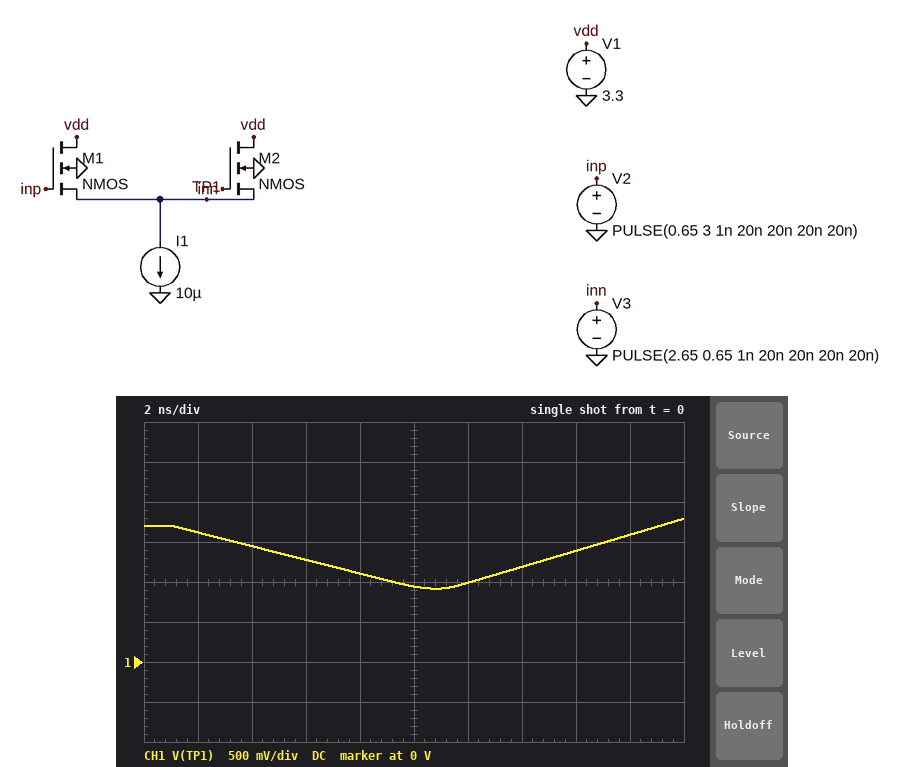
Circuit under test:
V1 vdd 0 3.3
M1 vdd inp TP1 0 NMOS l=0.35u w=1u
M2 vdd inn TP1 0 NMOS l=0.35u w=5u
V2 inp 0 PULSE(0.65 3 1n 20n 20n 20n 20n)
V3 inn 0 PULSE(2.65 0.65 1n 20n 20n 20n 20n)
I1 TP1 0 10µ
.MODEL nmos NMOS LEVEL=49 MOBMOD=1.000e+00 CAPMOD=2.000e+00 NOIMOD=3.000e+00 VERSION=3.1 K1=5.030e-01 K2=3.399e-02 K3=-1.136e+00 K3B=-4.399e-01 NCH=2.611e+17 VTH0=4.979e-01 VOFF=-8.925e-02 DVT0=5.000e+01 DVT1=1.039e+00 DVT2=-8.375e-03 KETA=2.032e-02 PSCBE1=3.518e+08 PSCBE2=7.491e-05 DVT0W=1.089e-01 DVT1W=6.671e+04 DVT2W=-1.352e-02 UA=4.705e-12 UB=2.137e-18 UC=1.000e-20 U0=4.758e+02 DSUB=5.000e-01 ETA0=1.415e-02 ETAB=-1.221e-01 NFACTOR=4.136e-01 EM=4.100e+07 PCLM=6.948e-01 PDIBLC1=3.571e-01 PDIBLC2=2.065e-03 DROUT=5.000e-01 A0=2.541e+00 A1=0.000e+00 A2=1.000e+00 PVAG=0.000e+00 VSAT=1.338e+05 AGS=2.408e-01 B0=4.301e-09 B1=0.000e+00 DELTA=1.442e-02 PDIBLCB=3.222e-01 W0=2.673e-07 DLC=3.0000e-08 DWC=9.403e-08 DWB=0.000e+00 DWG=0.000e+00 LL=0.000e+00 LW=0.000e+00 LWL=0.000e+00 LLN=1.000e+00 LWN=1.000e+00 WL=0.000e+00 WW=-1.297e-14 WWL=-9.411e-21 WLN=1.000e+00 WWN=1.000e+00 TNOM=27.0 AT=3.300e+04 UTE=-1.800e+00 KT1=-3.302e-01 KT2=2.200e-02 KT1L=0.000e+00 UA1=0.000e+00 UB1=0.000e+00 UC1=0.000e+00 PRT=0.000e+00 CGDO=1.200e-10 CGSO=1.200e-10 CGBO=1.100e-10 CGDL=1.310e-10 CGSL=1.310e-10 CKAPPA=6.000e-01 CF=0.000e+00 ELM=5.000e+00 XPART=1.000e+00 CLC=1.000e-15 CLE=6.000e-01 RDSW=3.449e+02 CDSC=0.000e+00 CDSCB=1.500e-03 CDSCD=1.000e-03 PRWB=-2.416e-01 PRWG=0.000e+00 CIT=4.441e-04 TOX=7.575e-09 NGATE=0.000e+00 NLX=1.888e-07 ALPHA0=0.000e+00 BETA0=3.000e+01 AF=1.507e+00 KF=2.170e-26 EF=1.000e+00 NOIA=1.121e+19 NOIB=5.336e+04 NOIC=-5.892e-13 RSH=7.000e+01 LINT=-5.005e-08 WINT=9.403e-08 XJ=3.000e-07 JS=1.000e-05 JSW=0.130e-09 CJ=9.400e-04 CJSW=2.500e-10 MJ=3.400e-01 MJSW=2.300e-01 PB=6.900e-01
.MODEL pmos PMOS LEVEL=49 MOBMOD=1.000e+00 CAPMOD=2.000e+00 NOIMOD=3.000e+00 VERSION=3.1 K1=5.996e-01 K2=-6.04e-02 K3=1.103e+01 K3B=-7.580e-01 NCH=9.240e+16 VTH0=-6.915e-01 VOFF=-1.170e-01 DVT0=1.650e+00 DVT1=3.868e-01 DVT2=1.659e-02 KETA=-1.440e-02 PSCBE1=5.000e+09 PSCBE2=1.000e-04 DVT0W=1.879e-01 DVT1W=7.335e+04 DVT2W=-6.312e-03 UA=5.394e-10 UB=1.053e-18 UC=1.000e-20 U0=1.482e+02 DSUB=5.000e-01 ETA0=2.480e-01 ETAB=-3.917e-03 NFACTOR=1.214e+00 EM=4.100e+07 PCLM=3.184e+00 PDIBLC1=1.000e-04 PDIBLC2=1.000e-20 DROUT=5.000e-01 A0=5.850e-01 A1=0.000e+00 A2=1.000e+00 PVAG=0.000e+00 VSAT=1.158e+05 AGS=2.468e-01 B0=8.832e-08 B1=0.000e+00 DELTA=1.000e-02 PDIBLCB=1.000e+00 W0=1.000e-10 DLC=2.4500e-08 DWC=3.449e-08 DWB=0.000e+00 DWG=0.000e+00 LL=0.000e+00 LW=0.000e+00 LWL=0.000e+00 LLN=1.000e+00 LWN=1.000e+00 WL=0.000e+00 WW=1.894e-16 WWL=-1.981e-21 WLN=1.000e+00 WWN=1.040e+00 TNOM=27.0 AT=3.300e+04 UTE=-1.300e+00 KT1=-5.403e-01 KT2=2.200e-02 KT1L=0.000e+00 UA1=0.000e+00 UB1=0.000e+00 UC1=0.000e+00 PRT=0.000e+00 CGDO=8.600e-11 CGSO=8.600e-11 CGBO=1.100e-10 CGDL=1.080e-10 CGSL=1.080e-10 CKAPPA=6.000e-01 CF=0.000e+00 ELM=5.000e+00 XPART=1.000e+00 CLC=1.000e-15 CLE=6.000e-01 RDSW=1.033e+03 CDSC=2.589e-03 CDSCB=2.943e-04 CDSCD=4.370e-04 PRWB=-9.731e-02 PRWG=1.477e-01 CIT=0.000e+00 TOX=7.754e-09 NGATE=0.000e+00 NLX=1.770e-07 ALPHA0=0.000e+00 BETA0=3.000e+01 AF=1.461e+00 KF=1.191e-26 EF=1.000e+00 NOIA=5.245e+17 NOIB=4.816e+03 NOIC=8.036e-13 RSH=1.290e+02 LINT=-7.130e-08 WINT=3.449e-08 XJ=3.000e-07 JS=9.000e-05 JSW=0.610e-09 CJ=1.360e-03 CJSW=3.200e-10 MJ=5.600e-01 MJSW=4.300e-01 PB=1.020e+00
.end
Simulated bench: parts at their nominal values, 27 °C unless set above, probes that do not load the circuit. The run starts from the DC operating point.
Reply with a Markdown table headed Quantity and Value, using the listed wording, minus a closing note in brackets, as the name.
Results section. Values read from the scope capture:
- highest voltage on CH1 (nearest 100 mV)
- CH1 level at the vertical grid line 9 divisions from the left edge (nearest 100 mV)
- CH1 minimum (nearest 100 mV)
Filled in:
| Quantity | Value |
|---|---|
| highest voltage on CH1 | 1.8 V |
| CH1 level at the vertical grid line 9 divisions from the left edge | 1.6 V |
| CH1 minimum | 900 mV |
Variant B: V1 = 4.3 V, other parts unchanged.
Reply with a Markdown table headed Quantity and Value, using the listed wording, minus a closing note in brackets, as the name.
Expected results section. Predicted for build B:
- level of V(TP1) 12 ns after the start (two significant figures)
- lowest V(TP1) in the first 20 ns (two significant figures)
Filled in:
| Quantity | Value |
|---|---|
| level of V(TP1) 12 ns after the start | 1.0 V |
| lowest V(TP1) in the first 20 ns | 930 mV |
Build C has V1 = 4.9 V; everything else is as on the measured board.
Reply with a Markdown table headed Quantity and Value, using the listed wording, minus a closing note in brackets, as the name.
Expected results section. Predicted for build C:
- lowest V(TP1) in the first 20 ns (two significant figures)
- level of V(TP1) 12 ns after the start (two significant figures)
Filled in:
| Quantity | Value |
|---|---|
| lowest V(TP1) in the first 20 ns | 950 mV |
| level of V(TP1) 12 ns after the start | 1.0 V |
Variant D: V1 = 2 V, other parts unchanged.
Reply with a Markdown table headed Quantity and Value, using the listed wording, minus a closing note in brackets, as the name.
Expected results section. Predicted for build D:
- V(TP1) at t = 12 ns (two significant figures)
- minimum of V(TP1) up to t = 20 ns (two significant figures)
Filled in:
| Quantity | Value |
|---|---|
| V(TP1) at t = 12 ns | 970 mV |
| minimum of V(TP1) up to t = 20 ns | 900 mV |
